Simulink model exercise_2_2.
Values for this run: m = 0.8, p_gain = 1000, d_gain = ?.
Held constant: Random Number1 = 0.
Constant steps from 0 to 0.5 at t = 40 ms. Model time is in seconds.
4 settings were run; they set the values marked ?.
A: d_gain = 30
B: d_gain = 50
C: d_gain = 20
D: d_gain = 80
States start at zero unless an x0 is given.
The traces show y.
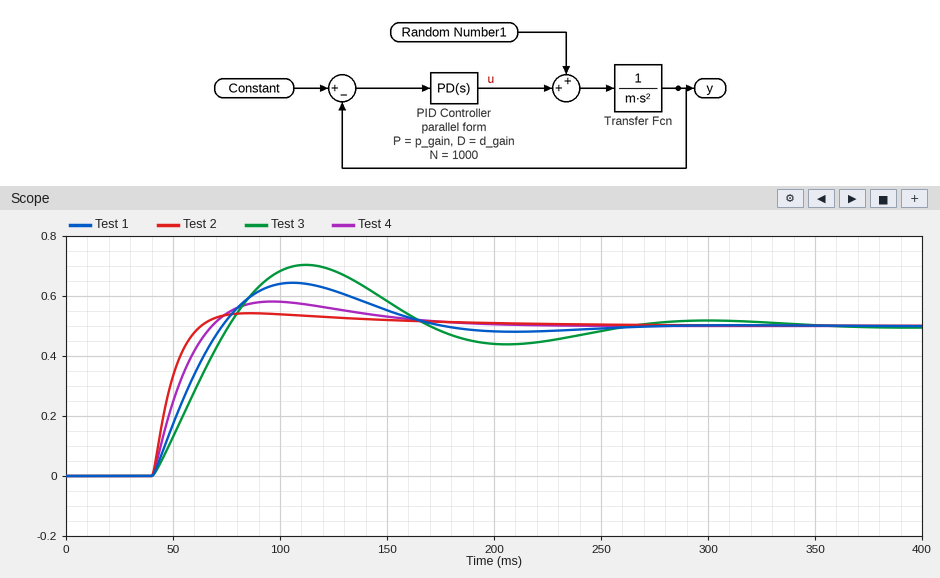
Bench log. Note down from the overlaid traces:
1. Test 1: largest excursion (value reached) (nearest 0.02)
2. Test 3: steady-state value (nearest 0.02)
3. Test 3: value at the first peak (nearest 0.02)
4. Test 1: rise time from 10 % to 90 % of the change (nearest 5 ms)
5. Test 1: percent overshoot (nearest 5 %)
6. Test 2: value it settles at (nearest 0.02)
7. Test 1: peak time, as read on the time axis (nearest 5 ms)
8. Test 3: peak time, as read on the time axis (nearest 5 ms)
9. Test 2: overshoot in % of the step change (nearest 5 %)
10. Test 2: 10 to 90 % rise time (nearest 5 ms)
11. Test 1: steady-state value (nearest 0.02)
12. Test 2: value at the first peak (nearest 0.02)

0.64
0.50
0.70
25 ms
30 %
0.50
105 ms
110 ms
10 %
15 ms
0.50
0.54
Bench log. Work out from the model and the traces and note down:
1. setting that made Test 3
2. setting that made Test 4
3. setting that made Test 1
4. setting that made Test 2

C
B
A
D
